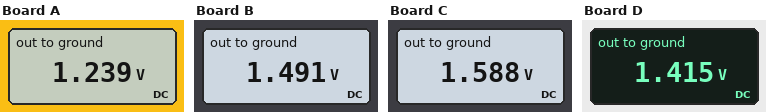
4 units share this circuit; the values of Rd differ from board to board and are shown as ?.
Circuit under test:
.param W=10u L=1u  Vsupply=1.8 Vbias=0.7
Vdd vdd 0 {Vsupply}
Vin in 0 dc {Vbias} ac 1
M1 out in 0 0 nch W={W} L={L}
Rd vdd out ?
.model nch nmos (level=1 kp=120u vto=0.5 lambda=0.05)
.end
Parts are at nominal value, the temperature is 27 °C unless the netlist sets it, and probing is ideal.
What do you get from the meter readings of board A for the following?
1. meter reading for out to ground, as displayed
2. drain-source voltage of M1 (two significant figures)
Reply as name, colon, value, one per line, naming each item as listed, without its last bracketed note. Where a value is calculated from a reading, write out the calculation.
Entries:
meter reading for out to ground, as displayed: 1.239 V
drain-source voltage of M1: 1.239 V = 1.2 V
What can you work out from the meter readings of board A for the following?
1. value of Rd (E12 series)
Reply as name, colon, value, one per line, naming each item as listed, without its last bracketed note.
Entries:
value of Rd: 22 kΩ
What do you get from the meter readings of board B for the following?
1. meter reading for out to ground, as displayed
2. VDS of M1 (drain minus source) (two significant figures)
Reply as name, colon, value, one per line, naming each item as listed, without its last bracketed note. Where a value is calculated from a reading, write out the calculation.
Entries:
meter reading for out to ground, as displayed: 1.491 V
VDS of M1 (drain minus source): 1.491 V = 1.5 V
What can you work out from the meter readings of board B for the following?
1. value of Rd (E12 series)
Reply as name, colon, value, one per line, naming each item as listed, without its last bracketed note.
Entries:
value of Rd: 12 kΩ
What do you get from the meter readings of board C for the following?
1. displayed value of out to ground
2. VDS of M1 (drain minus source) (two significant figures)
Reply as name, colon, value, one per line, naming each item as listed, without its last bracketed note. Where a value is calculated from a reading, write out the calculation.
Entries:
displayed value of out to ground: 1.588 V
VDS of M1 (drain minus source): 1.588 V = 1.6 V
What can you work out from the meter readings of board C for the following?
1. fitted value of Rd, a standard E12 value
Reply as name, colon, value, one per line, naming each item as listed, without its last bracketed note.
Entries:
fitted value of Rd, a standard E12 value: 8.2 kΩ
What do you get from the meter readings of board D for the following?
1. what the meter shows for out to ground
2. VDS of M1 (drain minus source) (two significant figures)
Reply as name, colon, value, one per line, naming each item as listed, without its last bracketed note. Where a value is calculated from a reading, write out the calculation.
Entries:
what the meter shows for out to ground: 1.415 V
VDS of M1 (drain minus source): 1.415 V = 1.4 V
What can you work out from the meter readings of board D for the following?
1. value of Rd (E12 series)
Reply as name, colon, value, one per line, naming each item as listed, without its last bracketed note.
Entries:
value of Rd: 15 kΩ
